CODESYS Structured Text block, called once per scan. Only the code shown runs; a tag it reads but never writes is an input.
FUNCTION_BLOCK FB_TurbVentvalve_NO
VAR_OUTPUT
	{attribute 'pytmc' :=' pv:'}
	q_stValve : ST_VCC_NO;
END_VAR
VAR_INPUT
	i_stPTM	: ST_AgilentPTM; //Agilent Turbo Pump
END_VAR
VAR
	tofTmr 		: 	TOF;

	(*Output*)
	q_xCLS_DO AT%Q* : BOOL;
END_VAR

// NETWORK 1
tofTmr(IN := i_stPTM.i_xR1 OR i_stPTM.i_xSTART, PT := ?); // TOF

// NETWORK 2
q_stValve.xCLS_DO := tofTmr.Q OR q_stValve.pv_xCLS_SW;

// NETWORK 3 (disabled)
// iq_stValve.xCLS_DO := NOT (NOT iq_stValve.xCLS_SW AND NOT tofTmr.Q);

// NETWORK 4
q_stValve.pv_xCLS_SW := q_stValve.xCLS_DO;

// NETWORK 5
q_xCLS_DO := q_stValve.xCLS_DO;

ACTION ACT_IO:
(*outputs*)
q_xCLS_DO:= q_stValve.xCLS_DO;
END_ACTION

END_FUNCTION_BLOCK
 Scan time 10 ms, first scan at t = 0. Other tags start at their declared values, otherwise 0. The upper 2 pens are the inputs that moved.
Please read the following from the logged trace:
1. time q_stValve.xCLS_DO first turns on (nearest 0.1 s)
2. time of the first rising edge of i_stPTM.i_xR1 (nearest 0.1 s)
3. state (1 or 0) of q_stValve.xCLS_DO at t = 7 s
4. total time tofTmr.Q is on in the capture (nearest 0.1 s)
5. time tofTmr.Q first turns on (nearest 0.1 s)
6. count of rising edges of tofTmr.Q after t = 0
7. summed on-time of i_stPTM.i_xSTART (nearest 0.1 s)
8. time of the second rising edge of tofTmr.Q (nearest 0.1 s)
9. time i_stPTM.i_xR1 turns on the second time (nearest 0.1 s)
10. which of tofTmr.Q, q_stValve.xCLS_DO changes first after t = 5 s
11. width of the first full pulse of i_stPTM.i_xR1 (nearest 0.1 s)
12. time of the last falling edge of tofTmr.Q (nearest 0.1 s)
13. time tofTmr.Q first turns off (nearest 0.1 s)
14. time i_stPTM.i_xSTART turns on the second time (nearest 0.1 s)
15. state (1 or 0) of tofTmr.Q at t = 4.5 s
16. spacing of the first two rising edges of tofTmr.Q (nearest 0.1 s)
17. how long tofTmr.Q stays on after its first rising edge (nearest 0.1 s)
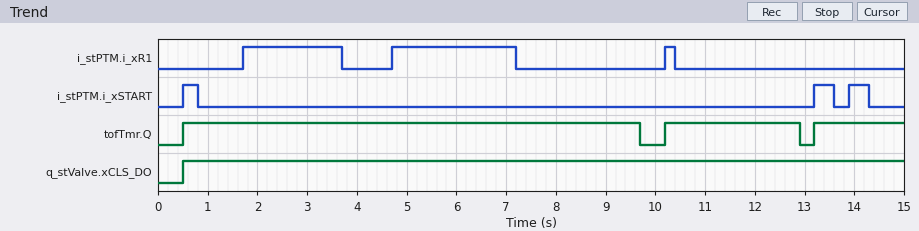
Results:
0.5 s
1.7 s
1
13.7 s
0.5 s
3
1.1 s
10.2 s
4.7 s
tofTmr.Q
2.0 s
12.9 s
9.7 s
13.2 s
1
9.7 s
9.2 s
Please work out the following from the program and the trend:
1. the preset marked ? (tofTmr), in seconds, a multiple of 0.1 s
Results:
2.5 s
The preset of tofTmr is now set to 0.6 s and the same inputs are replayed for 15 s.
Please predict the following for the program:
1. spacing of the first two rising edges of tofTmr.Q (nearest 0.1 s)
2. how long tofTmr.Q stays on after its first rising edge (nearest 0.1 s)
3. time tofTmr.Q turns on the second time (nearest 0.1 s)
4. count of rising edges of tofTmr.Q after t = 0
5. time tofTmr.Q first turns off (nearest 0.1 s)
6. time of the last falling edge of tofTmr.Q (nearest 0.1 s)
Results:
1.2 s
0.9 s
1.7 s
5
1.4 s
14.9 s
